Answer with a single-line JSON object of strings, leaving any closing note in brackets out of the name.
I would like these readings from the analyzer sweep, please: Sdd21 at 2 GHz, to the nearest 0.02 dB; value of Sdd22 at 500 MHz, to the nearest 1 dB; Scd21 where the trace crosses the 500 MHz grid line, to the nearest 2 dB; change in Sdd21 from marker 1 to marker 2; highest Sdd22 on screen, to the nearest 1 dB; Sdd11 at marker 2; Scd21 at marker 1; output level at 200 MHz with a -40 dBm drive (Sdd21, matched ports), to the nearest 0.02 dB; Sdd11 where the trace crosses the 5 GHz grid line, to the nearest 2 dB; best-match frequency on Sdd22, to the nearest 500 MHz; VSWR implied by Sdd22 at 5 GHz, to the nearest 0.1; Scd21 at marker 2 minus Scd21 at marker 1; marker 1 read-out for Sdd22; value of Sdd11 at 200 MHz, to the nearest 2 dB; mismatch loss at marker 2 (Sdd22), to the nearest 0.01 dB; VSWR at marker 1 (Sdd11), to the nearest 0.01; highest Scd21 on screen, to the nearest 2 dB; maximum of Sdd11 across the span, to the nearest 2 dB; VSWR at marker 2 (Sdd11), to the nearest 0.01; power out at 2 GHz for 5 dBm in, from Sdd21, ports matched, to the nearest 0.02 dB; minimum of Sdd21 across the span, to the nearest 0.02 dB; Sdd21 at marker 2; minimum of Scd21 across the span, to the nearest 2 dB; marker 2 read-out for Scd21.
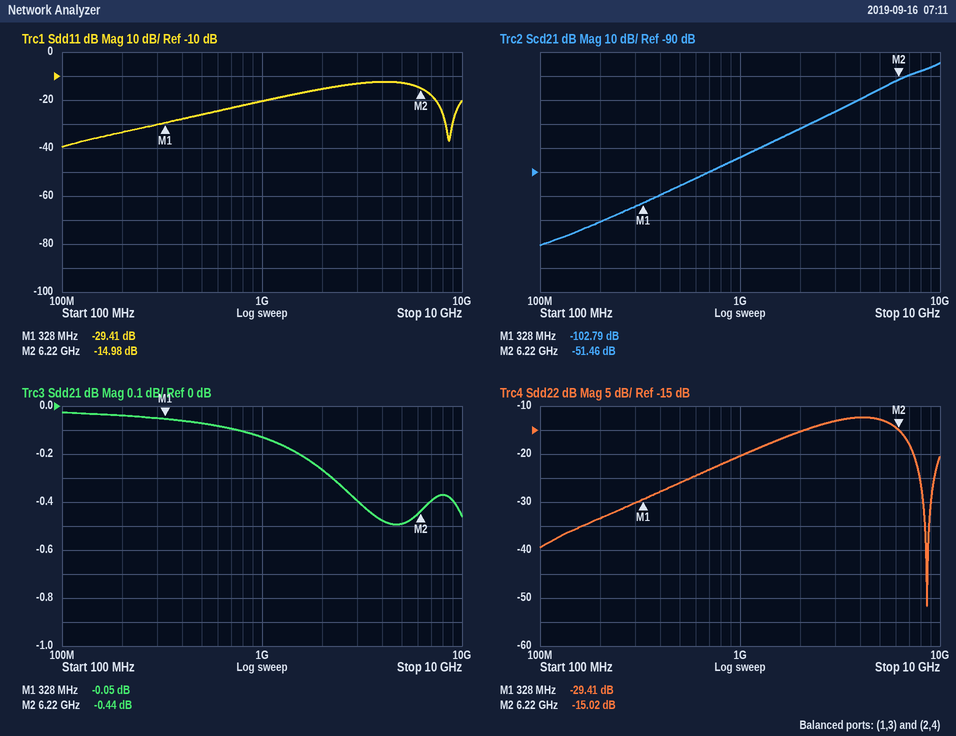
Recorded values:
{"Sdd21 at 2 GHz, to the nearest 0.02 dB": "-0.26 dB", "value of Sdd22 at 500 MHz, to the nearest 1 dB": "-26 dB", "Scd21 where the trace crosses the 500 MHz grid line, to the nearest 2 dB": "-96 dB", "change in Sdd21 from marker 1 to marker 2": "-0.39 dB", "highest Sdd22 on screen, to the nearest 1 dB": "-12 dB", "Sdd11 at marker 2": "-14.98 dB", "Scd21 at marker 1": "-102.79 dB", "output level at 200 MHz with a -40 dBm drive (Sdd21, matched ports), to the nearest 0.02 dB": "-40.04 dBm", "Sdd11 where the trace crosses the 5 GHz grid line, to the nearest 2 dB": "-12 dB", "best-match frequency on Sdd22, to the nearest 500 MHz": "8.5 GHz", "VSWR implied by Sdd22 at 5 GHz, to the nearest 0.1": "1.6", "Scd21 at marker 2 minus Scd21 at marker 1": "51.33 dB", "marker 1 read-out for Sdd22": "-29.41 dB", "value of Sdd11 at 200 MHz, to the nearest 2 dB": "-34 dB", "mismatch loss at marker 2 (Sdd22), to the nearest 0.01 dB": "0.14 dB", "VSWR at marker 1 (Sdd11), to the nearest 0.01": "1.07", "highest Scd21 on screen, to the nearest 2 dB": "-44 dB", "maximum of Sdd11 across the span, to the nearest 2 dB": "-12 dB", "VSWR at marker 2 (Sdd11), to the nearest 0.01": "1.43", "power out at 2 GHz for 5 dBm in, from Sdd21, ports matched, to the nearest 0.02 dB": "4.74 dBm", "minimum of Sdd21 across the span, to the nearest 0.02 dB": "-0.50 dB", "Sdd21 at marker 2": "-0.44 dB", "minimum of Scd21 across the span, to the nearest 2 dB": "-120 dB", "marker 2 read-out for Scd21": "-51.46 dB"}
